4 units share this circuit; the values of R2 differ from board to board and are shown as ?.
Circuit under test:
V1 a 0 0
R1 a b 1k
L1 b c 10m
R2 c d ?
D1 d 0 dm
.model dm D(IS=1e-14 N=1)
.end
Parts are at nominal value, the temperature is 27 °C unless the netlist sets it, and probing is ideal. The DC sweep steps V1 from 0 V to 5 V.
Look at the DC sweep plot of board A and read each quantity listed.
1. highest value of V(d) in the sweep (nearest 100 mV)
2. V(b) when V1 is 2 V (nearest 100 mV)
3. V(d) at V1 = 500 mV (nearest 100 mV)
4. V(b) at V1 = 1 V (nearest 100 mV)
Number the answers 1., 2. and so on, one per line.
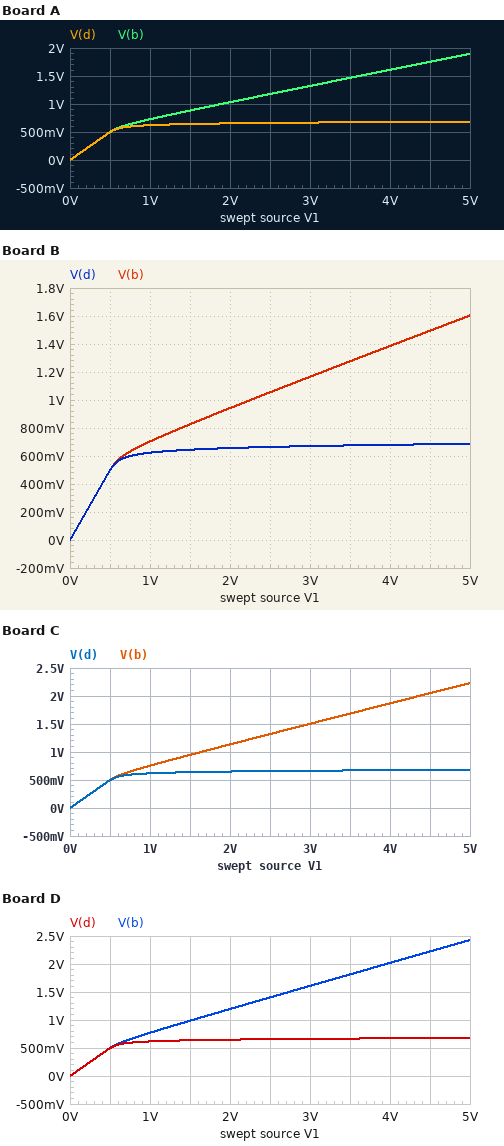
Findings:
1. 700 mV
2. 1.0 V
3. 500 mV
4. 700 mV
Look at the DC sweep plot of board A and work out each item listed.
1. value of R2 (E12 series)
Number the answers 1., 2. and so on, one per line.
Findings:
1. 390 Ω
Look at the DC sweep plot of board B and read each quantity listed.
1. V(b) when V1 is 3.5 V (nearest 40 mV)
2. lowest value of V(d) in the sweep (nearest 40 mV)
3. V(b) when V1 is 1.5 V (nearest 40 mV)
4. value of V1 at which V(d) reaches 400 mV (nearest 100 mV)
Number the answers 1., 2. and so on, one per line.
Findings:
1. 1.28 V
2. 0 V
3. 840 mV
4. 400 mV
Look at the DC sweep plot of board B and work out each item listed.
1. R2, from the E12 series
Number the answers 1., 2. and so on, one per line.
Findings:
1. 270 Ω
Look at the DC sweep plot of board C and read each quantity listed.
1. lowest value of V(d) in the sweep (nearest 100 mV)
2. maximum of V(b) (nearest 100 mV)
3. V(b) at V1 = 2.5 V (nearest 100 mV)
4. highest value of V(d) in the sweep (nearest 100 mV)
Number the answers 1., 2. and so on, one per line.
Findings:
1. 0 V
2. 2.2 V
3. 1.3 V
4. 700 mV
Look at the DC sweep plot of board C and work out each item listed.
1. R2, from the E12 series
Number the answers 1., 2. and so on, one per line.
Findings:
1. 560 Ω
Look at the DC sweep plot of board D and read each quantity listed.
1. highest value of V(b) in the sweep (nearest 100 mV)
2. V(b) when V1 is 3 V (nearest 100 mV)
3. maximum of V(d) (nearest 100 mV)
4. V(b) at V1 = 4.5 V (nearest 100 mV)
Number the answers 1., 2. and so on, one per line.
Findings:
1. 2.4 V
2. 1.6 V
3. 700 mV
4. 2.2 V
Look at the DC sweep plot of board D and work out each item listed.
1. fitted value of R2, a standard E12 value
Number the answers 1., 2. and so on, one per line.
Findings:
1. 680 Ω
